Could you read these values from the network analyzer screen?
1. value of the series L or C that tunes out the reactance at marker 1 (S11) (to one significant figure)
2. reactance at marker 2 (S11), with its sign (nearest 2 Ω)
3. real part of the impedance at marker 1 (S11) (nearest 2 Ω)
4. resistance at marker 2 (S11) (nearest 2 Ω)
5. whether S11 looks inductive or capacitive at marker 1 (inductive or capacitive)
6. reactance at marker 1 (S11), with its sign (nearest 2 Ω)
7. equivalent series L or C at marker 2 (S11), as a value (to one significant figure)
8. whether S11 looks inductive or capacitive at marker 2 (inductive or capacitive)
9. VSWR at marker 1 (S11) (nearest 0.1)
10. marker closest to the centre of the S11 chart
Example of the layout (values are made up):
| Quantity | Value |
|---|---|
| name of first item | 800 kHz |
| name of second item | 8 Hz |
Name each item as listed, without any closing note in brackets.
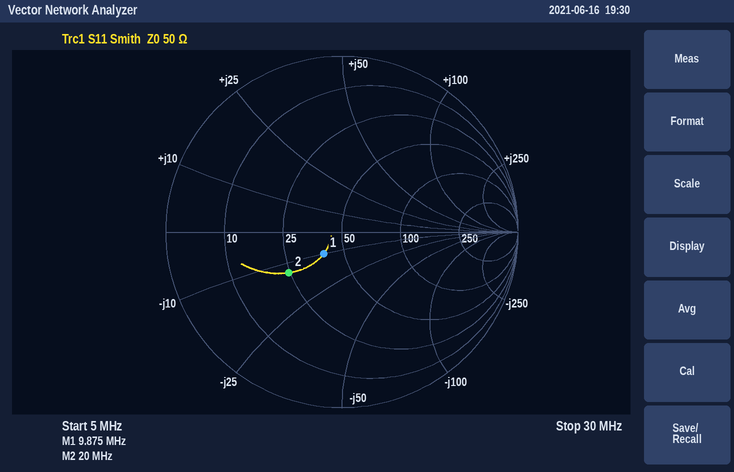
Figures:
| Quantity | Value |
|---|---|
| value of the series L or C that tunes out the reactance at marker 1 (S11) | 200 nH |
| reactance at marker 2 (S11), with its sign | -14 Ω |
| real part of the impedance at marker 1 (S11) | 40 Ω |
| resistance at marker 2 (S11) | 24 Ω |
| whether S11 looks inductive or capacitive at marker 1 | capacitive |
| reactance at marker 1 (S11), with its sign | -10 Ω |
| equivalent series L or C at marker 2 (S11), as a value | 600 pF |
| whether S11 looks inductive or capacitive at marker 2 | capacitive |
| VSWR at marker 1 (S11) | 1.4 |
| marker closest to the centre of the S11 chart | marker 1 |
